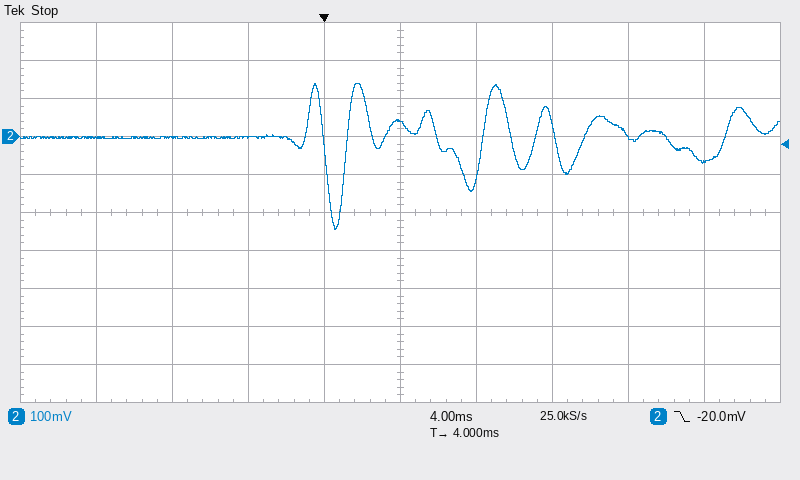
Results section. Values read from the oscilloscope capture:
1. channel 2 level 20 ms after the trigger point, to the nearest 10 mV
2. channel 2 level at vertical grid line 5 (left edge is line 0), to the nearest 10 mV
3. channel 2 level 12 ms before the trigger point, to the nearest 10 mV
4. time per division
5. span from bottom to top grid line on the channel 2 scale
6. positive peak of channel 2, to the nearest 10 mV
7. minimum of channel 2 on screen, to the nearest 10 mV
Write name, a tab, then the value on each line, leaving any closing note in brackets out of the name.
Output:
channel 2 level 20 ms after the trigger point, to the nearest 10 mV	-70 mV
channel 2 level at vertical grid line 5 (left edge is line 0), to the nearest 10 mV	40 mV
channel 2 level 12 ms before the trigger point, to the nearest 10 mV	0 mV
time per division	4 ms
span from bottom to top grid line on the channel 2 scale	1 V
positive peak of channel 2, to the nearest 10 mV	140 mV
minimum of channel 2 on screen, to the nearest 10 mV	-240 mV
